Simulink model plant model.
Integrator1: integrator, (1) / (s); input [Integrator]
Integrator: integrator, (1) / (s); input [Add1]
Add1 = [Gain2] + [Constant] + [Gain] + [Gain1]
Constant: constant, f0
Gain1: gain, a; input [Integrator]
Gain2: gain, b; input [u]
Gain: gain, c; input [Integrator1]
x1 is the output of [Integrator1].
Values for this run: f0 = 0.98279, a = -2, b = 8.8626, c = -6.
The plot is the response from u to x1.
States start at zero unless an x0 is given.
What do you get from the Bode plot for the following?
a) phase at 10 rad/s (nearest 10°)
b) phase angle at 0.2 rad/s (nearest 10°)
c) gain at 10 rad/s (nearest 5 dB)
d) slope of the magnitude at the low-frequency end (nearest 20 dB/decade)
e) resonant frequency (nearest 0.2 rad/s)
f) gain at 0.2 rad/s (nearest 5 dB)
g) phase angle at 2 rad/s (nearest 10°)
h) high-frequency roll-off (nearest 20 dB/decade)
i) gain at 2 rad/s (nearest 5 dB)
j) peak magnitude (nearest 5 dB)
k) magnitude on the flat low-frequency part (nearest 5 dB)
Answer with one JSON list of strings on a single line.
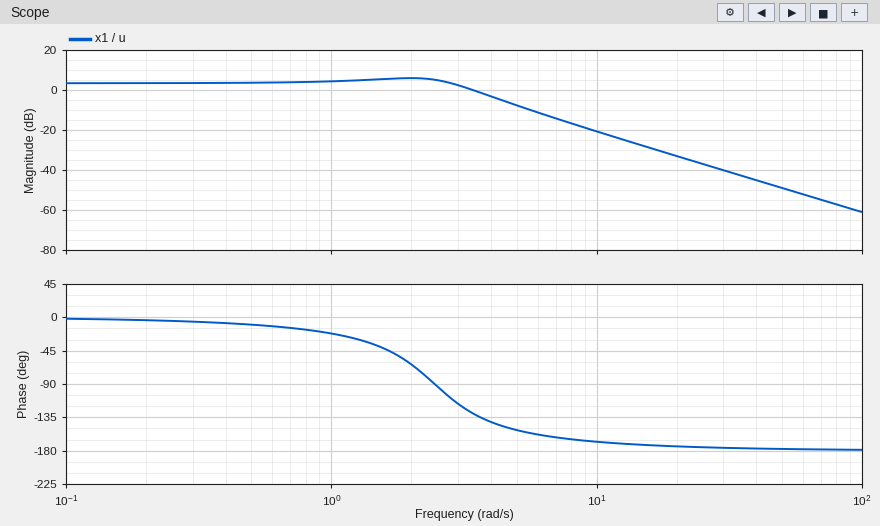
["-170°", "0°", "-20 dB", "0 dB/decade", "2.0 rad/s", "5 dB", "-60°", "-40 dB/decade", "5 dB", "5 dB", "5 dB"]
